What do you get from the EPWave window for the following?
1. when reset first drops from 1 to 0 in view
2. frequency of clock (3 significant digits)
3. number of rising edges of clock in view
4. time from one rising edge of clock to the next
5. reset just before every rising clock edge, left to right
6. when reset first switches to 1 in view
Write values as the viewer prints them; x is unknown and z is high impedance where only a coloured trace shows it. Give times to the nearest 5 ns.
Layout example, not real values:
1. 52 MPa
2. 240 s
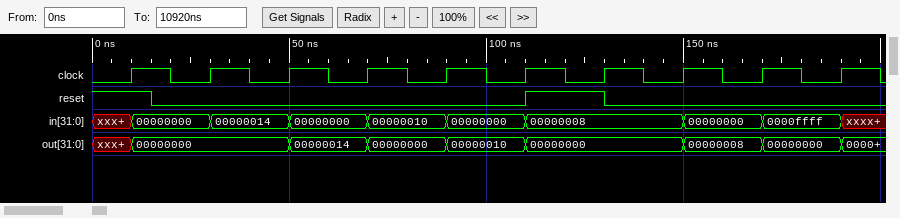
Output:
1. 15 ns
2. 50.0 MHz
3. 10
4. 20 ns
5. 1 0 0 0 0 0 1 0 0 0
6. 110 ns
